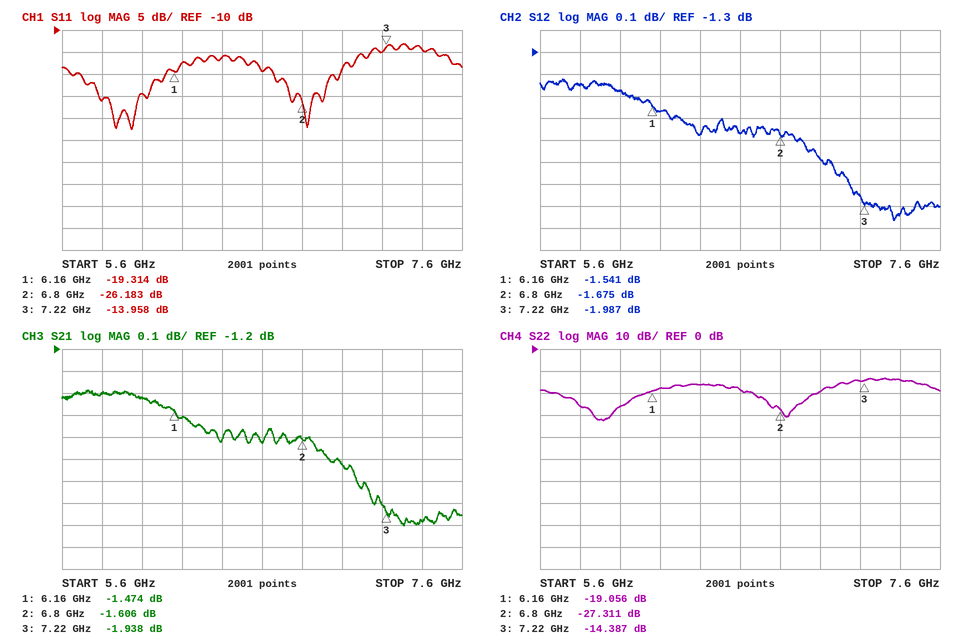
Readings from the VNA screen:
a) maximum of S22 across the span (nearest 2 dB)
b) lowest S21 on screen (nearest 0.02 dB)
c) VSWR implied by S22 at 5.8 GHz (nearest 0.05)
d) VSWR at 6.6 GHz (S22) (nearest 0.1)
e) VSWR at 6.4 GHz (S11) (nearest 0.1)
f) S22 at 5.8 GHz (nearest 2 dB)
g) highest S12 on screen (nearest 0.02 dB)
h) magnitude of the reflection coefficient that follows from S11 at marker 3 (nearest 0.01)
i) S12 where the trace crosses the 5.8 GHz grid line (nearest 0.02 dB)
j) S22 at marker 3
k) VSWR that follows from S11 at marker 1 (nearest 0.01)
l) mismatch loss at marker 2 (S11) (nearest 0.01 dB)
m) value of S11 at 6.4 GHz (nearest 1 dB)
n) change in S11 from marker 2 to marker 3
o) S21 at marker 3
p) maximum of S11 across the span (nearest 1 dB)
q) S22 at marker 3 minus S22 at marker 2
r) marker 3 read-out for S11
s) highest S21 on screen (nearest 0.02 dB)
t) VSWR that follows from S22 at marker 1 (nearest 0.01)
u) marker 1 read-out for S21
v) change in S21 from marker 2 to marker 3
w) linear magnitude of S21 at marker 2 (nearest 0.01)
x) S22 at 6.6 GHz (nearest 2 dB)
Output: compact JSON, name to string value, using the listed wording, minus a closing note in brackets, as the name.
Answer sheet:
{"maximum of S22 across the span": "-14 dB", "lowest S21 on screen": "-2.00 dB", "VSWR implied by S22 at 5.8 GHz": "1.10", "VSWR at 6.6 GHz (S22)": "1.3", "VSWR at 6.4 GHz (S11)": "1.4", "S22 at 5.8 GHz": "-26 dB", "highest S12 on screen": "-1.42 dB", "magnitude of the reflection coefficient that follows from S11 at marker 3": "0.20", "S12 where the trace crosses the 5.8 GHz grid line": "-1.44 dB", "S22 at marker 3": "-14.387 dB", "VSWR that follows from S11 at marker 1": "1.24", "mismatch loss at marker 2 (S11)": "0.01 dB", "value of S11 at 6.4 GHz": "-16 dB", "change in S11 from marker 2 to marker 3": "12.225 dB", "S21 at marker 3": "-1.938 dB", "maximum of S11 across the span": "-13 dB", "S22 at marker 3 minus S22 at marker 2": "12.924 dB", "marker 3 read-out for S11": "-13.958 dB", "highest S21 on screen": "-1.38 dB", "VSWR that follows from S22 at marker 1": "1.25", "marker 1 read-out for S21": "-1.474 dB", "change in S21 from marker 2 to marker 3": "-0.332 dB", "linear magnitude of S21 at marker 2": "0.83", "S22 at 6.6 GHz": "-18 dB"}
